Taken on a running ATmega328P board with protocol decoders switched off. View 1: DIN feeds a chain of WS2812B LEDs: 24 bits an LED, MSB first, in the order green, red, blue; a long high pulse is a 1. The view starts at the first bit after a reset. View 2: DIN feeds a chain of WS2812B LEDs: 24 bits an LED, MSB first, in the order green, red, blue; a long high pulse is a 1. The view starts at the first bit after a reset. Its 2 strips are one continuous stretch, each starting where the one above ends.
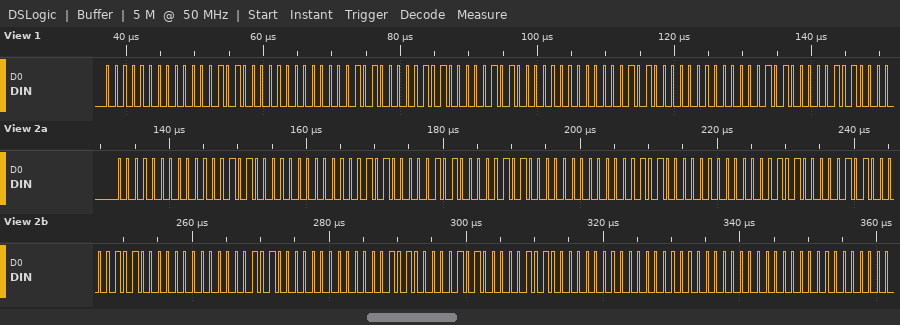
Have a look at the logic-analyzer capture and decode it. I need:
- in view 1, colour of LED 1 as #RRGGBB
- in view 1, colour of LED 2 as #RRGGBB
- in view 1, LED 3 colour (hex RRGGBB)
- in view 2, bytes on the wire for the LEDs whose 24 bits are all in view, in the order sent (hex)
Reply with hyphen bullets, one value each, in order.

- #050000
- #050505
- #050000
- 00 05 00 05 05 05 00 05 00 05 05 05 00 05 00 05 05 05 00 00 00
